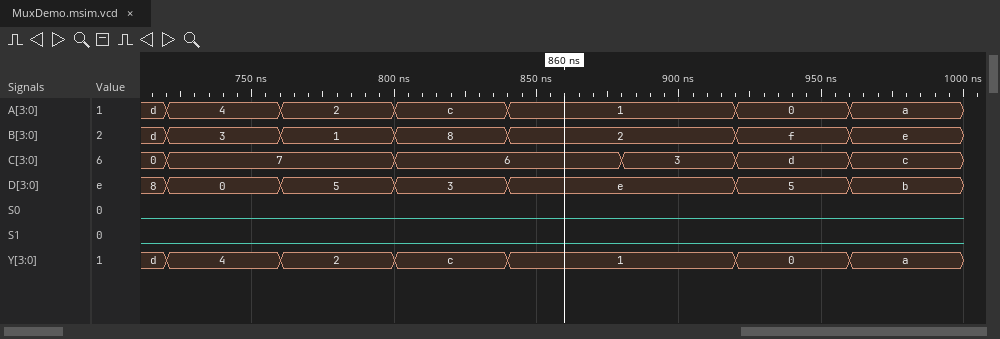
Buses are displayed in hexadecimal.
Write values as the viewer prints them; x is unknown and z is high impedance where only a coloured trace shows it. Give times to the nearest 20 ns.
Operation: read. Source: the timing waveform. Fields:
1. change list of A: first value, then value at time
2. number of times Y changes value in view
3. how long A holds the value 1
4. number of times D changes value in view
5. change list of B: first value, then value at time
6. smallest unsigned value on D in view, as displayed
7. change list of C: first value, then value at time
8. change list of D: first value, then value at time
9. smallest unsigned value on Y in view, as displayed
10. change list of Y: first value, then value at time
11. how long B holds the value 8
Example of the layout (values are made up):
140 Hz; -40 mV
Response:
d, 4 at 720 ns, 2 at 760 ns, c at 800 ns, 1 at 840 ns, 0 at 920 ns, a at 960 ns; 6; 80 ns; 6; d, 3 at 720 ns, 1 at 760 ns, 8 at 800 ns, 2 at 840 ns, f at 920 ns, e at 960 ns; 0; 0, 7 at 720 ns, 6 at 800 ns, 3 at 880 ns, d at 920 ns, c at 960 ns; 8, 0 at 720 ns, 5 at 760 ns, 3 at 800 ns, e at 840 ns, 5 at 920 ns, b at 960 ns; 0; d, 4 at 720 ns, 2 at 760 ns, c at 800 ns, 1 at 840 ns, 0 at 920 ns, a at 960 ns; 40 ns
